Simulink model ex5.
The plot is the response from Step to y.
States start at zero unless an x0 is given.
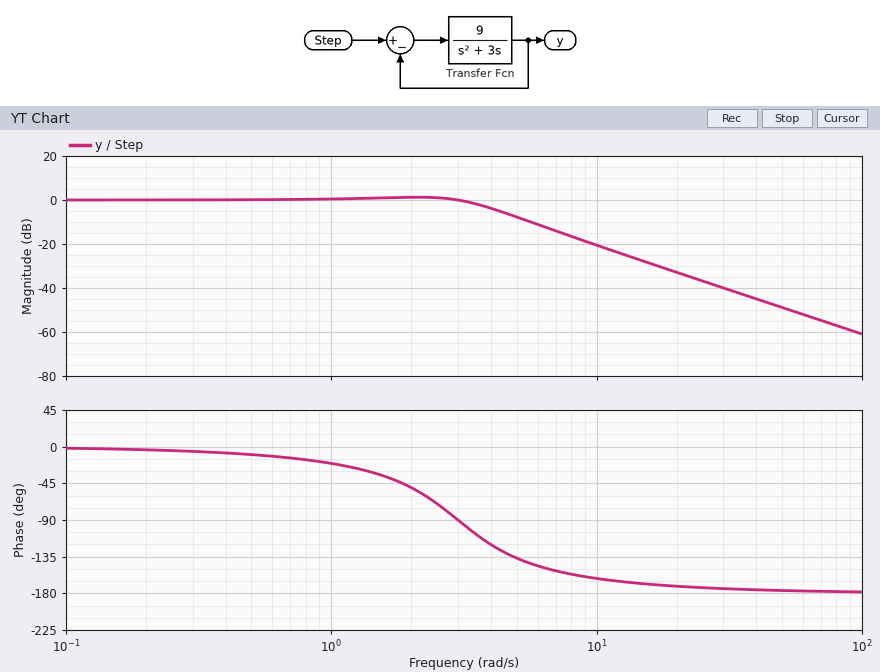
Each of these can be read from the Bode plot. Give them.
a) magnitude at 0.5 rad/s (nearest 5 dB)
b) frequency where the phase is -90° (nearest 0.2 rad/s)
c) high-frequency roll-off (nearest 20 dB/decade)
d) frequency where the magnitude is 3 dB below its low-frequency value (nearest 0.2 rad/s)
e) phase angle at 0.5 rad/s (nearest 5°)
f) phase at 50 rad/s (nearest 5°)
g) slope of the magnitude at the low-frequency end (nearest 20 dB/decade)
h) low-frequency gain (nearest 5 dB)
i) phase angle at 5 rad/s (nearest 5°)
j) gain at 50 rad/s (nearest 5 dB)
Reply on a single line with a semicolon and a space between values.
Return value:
0 dB; 3.0 rad/s; -40 dB/decade; 3.8 rad/s; -10°; -175°; 0 dB/decade; 0 dB; -135°; -50 dB
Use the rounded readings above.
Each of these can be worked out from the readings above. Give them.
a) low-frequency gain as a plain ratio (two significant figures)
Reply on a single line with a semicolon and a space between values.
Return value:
1.0
